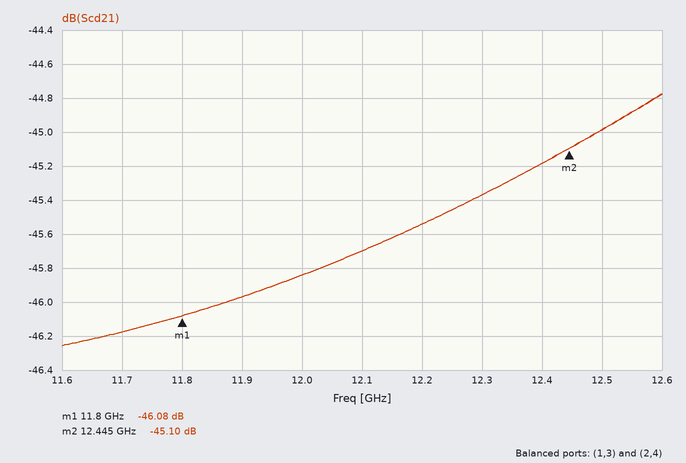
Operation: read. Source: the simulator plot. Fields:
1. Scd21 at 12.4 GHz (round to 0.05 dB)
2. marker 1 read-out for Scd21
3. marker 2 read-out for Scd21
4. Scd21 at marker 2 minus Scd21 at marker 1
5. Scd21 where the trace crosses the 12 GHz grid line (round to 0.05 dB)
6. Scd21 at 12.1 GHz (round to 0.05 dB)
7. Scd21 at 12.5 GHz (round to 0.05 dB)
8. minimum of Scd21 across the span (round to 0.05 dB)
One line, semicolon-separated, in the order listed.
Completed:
-45.20 dB; -46.08 dB; -45.10 dB; 0.98 dB; -45.85 dB; -45.70 dB; -45.00 dB; -46.25 dB
